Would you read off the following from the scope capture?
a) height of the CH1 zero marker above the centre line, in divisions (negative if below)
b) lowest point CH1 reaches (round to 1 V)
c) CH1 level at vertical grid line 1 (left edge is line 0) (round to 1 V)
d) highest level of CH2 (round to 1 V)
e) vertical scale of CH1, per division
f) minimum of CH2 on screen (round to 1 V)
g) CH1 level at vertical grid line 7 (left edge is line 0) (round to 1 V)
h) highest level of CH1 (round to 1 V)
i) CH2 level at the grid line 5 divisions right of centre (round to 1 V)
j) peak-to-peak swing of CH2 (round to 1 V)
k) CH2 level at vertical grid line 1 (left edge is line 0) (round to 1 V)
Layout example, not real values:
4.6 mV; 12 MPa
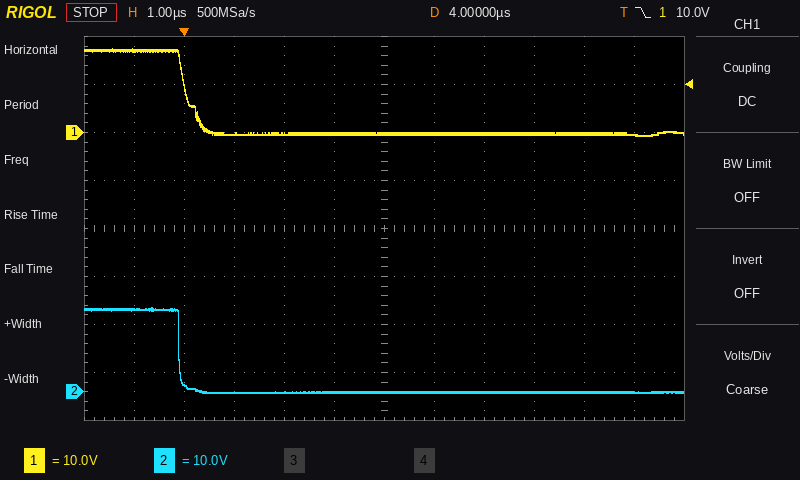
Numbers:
+2.0 div; -1 V; 17 V; 18 V; 10 V; 0 V; 0 V; 18 V; 0 V; 18 V; 17 V
